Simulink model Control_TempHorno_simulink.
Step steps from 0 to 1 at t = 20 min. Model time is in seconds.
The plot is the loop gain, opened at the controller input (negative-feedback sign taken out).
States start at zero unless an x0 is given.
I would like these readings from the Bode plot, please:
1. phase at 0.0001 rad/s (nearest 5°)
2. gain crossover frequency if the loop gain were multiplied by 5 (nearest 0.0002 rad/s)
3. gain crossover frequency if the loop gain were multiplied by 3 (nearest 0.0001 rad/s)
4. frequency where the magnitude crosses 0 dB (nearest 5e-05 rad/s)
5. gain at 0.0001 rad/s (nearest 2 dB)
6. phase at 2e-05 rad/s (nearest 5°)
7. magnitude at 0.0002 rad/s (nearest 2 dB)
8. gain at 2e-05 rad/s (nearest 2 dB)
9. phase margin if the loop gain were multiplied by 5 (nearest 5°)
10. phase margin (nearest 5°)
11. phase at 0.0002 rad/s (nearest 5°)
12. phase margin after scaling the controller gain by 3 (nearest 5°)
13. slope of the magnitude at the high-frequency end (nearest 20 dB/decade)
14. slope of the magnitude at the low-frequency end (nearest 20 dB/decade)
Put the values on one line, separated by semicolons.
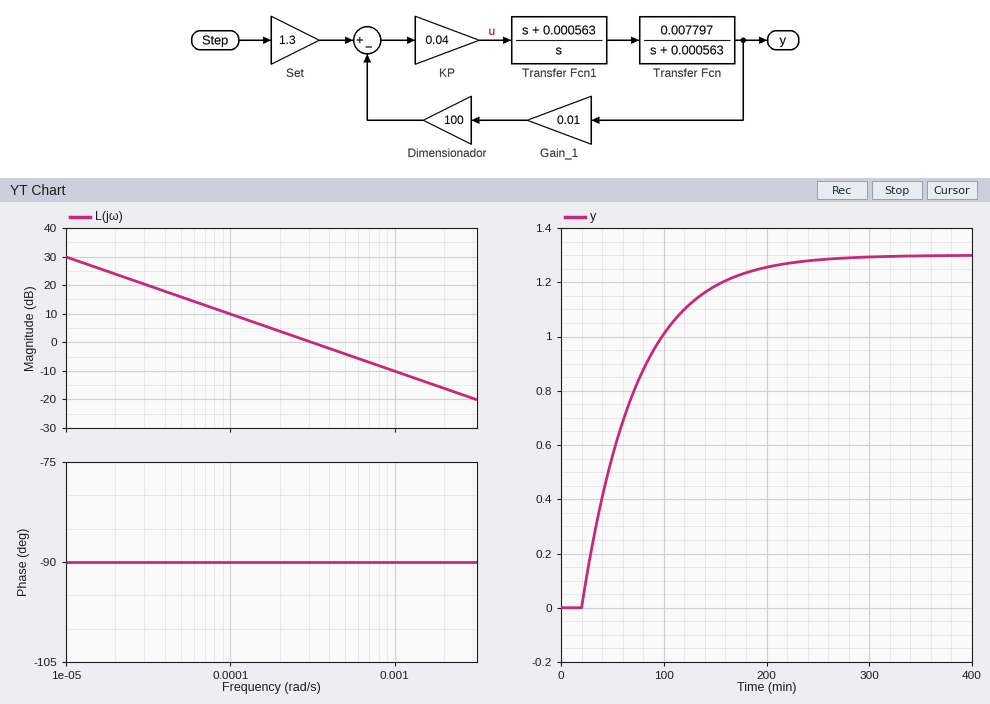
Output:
-90°; 0.0016 rad/s; 0.0009 rad/s; 0.00030 rad/s; 10 dB; -90°; 4 dB; 24 dB; 90°; 90°; -90°; 90°; -20 dB/decade; -20 dB/decade
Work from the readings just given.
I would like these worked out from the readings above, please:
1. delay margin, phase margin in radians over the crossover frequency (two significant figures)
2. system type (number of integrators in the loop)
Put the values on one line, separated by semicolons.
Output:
5200 s; 1
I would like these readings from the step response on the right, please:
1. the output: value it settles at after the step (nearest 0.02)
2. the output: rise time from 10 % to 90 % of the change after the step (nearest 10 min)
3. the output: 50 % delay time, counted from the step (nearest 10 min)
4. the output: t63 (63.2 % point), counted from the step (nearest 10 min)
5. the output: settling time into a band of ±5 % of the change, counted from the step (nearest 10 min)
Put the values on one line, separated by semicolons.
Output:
1.30; 120 min; 40 min; 50 min; 160 min
